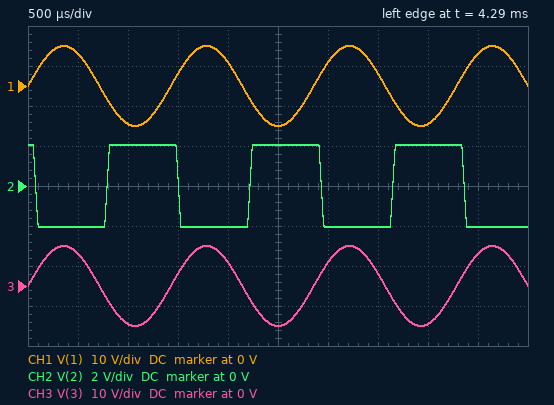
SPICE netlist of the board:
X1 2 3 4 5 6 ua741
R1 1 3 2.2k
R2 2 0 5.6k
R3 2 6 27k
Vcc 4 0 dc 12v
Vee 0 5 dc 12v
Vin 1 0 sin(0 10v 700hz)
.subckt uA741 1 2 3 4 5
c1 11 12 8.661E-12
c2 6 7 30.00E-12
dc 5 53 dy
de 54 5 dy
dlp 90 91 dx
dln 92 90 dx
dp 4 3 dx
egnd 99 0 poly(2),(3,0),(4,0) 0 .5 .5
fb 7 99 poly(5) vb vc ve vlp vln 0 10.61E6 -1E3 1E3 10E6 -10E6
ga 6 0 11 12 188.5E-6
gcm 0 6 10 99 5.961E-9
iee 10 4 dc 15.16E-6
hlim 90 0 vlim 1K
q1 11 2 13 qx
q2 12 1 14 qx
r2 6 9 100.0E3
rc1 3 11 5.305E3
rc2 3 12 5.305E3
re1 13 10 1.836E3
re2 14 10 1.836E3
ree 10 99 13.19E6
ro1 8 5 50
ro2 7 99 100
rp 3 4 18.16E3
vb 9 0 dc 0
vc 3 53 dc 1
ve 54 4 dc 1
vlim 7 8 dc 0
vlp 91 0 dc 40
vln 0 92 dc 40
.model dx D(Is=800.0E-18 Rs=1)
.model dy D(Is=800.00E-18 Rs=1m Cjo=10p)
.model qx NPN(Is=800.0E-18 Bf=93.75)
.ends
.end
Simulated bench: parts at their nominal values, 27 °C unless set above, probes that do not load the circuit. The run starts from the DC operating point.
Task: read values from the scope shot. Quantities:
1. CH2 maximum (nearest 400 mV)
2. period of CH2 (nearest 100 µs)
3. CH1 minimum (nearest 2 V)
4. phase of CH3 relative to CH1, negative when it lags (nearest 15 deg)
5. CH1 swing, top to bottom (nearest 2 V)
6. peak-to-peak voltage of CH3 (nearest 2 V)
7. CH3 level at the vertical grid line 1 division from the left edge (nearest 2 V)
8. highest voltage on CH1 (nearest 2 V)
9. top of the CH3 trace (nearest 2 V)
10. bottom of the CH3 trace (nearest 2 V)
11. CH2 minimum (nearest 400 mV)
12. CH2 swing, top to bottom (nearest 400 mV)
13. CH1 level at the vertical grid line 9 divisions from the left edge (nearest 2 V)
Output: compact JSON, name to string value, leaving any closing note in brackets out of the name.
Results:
{"CH2 maximum": "2.0 V", "period of CH2": "1.4 ms", "CH1 minimum": "-10 V", "phase of CH3 relative to CH1, negative when it lags": "0 deg", "CH1 swing, top to bottom": "20 V", "peak-to-peak voltage of CH3": "20 V", "CH3 level at the vertical grid line 1 division from the left edge": "8 V", "highest voltage on CH1": "10 V", "top of the CH3 trace": "10 V", "bottom of the CH3 trace": "-10 V", "CH2 minimum": "-2.0 V", "CH2 swing, top to bottom": "4.0 V", "CH1 level at the vertical grid line 9 divisions from the left edge": "8 V"}
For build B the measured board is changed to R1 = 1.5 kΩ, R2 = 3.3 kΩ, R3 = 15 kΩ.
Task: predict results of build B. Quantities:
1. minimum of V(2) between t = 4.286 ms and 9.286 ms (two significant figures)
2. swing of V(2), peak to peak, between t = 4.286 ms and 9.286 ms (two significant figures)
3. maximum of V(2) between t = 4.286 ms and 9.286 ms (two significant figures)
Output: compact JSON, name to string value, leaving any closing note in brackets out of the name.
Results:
{"minimum of V(2) between t = 4.286 ms and 9.286 ms": "-2.1 V", "swing of V(2), peak to peak, between t = 4.286 ms and 9.286 ms": "4.3 V", "maximum of V(2) between t = 4.286 ms and 9.286 ms": "2.1 V"}
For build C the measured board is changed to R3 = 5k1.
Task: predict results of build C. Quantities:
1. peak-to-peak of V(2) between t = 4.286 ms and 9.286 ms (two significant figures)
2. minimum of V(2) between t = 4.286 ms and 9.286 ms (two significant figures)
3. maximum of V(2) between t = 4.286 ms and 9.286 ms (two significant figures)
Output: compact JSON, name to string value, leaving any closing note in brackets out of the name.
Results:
{"peak-to-peak of V(2) between t = 4.286 ms and 9.286 ms": "12 V", "minimum of V(2) between t = 4.286 ms and 9.286 ms": "-6.2 V", "maximum of V(2) between t = 4.286 ms and 9.286 ms": "6.2 V"}
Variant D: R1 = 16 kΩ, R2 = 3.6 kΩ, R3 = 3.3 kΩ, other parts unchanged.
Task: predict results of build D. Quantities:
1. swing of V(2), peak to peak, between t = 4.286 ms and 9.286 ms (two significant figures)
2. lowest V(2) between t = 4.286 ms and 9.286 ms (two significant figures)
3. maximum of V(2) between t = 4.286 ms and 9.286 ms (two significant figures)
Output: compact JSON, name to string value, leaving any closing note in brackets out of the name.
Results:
{"swing of V(2), peak to peak, between t = 4.286 ms and 9.286 ms": "12 V", "lowest V(2) between t = 4.286 ms and 9.286 ms": "-6.2 V", "maximum of V(2) between t = 4.286 ms and 9.286 ms": "6.2 V"}
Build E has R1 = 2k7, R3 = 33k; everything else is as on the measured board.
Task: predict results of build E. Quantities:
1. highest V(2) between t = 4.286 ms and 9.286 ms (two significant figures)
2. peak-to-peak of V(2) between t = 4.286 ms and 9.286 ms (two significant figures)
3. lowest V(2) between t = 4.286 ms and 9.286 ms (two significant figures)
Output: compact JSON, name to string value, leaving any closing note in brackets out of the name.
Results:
{"highest V(2) between t = 4.286 ms and 9.286 ms": "1.7 V", "peak-to-peak of V(2) between t = 4.286 ms and 9.286 ms": "3.4 V", "lowest V(2) between t = 4.286 ms and 9.286 ms": "-1.7 V"}
